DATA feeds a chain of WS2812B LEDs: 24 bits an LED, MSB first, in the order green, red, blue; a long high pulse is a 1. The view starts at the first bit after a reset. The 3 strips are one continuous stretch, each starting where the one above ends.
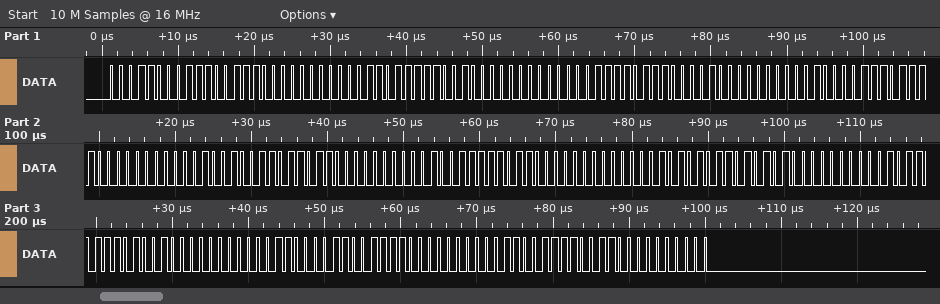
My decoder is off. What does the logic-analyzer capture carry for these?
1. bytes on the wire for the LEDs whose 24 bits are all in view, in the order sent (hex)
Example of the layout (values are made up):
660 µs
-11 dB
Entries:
18 E7 00 1B E4 00 1E E1 00 21 DE 00 24 DB 00 27 D8 00 2A D5 00 2D D2 00 30 CF 00 33 CC 00
